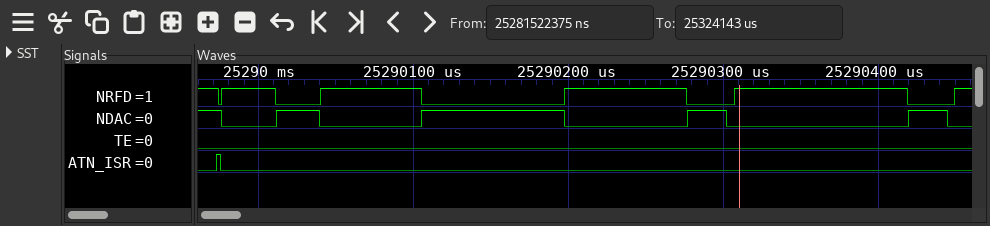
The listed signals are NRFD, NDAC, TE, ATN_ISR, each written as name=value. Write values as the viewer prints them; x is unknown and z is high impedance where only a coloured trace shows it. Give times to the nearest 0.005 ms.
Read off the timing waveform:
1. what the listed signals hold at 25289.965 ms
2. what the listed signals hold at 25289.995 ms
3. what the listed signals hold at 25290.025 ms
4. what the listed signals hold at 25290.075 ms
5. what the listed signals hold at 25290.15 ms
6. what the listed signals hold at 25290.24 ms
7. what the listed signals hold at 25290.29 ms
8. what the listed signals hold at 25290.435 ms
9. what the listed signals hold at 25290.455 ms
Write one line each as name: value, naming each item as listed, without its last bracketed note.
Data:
what the listed signals hold at 25289.965 ms: NRFD=1, NDAC=1, TE=0, ATN_ISR=0
what the listed signals hold at 25289.995 ms: NRFD=1, NDAC=0, TE=0, ATN_ISR=0
what the listed signals hold at 25290.025 ms: NRFD=0, NDAC=1, TE=0, ATN_ISR=0
what the listed signals hold at 25290.075 ms: NRFD=1, NDAC=0, TE=0, ATN_ISR=0
what the listed signals hold at 25290.15 ms: NRFD=0, NDAC=1, TE=0, ATN_ISR=0
what the listed signals hold at 25290.24 ms: NRFD=1, NDAC=0, TE=0, ATN_ISR=0
what the listed signals hold at 25290.29 ms: NRFD=0, NDAC=1, TE=0, ATN_ISR=0
what the listed signals hold at 25290.435 ms: NRFD=0, NDAC=1, TE=0, ATN_ISR=0
what the listed signals hold at 25290.455 ms: NRFD=1, NDAC=0, TE=0, ATN_ISR=0
